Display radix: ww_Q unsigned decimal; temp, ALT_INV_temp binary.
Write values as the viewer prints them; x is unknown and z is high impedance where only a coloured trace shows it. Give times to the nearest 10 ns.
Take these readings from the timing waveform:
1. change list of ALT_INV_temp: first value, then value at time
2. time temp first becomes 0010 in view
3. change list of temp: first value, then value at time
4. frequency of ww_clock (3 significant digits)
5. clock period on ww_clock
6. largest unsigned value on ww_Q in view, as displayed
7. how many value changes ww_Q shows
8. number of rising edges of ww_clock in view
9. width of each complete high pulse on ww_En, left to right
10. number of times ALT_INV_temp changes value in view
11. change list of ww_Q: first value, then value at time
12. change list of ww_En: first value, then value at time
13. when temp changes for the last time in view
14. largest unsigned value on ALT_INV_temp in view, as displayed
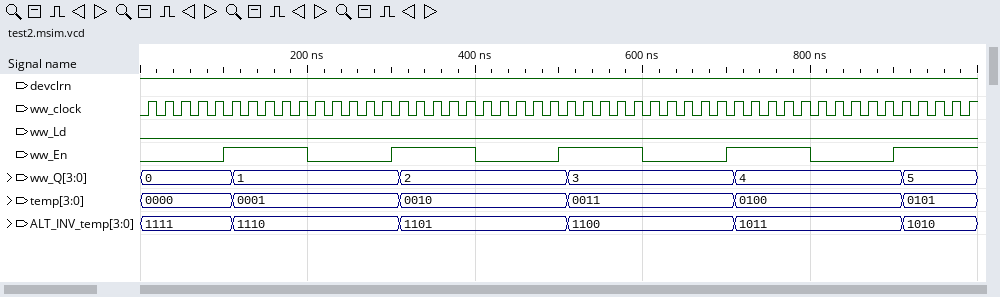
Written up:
1111, 1110 at 110 ns, 1101 at 310 ns, 1100 at 510 ns, 1011 at 710 ns, 1010 at 910 ns
310 ns
0000, 0001 at 110 ns, 0010 at 310 ns, 0011 at 510 ns, 0100 at 710 ns, 0101 at 910 ns
50.0 MHz
20 ns
5
5
50
100 ns, 100 ns, 100 ns, 100 ns
5
0, 1 at 110 ns, 2 at 310 ns, 3 at 510 ns, 4 at 710 ns, 5 at 910 ns
0, 1 at 100 ns, 0 at 200 ns, 1 at 300 ns, 0 at 400 ns, 1 at 500 ns, 0 at 600 ns, 1 at 700 ns, 0 at 800 ns, 1 at 900 ns
910 ns
1111
